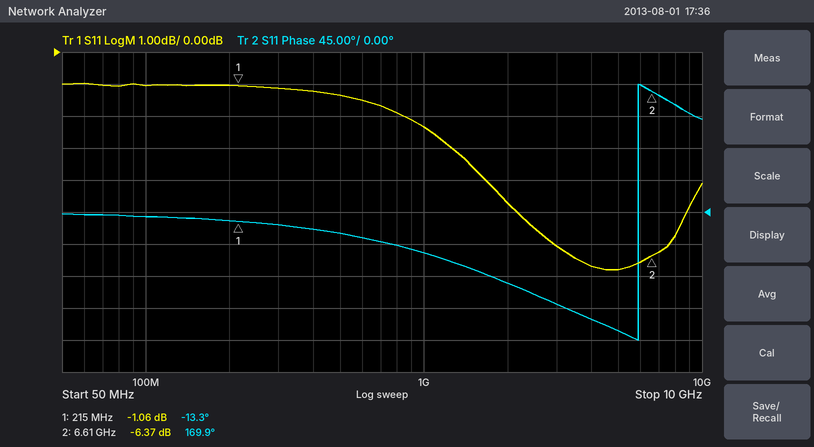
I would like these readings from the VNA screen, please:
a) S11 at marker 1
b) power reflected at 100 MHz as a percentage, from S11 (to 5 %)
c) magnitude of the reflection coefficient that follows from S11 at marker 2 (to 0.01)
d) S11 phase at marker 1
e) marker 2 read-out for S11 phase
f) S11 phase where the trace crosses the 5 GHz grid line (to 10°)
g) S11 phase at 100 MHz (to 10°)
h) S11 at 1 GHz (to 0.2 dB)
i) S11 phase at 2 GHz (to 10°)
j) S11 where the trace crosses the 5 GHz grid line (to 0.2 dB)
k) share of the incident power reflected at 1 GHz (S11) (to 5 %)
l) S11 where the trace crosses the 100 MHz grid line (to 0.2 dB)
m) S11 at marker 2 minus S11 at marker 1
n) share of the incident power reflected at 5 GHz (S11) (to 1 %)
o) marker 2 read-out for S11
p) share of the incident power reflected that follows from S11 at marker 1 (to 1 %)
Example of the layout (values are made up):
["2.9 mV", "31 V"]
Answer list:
["-1.06 dB", "80 %", "0.48", "-13.3°", "169.9°", "-170°", "-10°", "-2.4 dB", "-100°", "-6.8 dB", "60 %", "-1.0 dB", "-5.31 dB", "21 %", "-6.37 dB", "78 %"]
